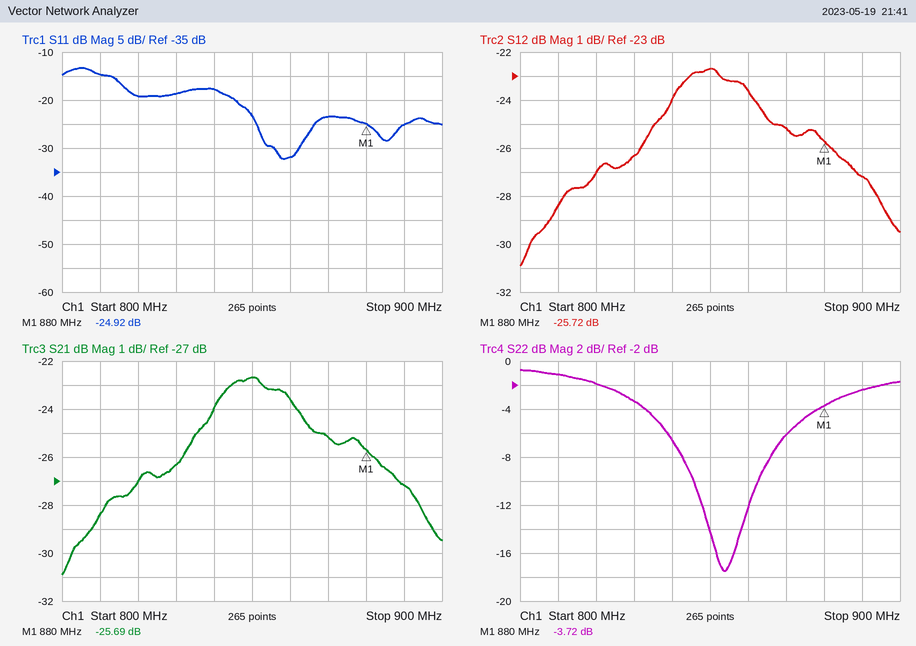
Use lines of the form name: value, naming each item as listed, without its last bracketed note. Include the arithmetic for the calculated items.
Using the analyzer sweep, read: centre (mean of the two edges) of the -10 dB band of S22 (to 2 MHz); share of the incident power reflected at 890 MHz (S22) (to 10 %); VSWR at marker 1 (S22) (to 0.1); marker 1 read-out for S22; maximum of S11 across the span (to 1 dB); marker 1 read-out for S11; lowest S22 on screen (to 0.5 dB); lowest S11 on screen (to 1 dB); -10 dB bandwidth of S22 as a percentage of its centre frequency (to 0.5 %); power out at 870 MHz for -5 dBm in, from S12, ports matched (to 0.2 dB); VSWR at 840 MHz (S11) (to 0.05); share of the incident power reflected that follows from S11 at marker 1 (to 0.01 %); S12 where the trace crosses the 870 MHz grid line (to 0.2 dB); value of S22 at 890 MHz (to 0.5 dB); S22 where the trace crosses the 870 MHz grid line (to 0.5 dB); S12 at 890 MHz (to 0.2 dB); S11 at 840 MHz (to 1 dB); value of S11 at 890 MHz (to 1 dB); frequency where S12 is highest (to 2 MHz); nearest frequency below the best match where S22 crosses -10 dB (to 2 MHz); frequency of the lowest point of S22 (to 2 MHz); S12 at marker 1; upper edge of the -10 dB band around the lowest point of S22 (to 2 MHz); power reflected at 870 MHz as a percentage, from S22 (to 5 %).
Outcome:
centre (mean of the two edges) of the -10 dB band of S22: 854 MHz
share of the incident power reflected at 890 MHz (S22): 10^(-2.5/10) ≈ 56.2 %, so 60 % to the nearest 10 %
VSWR at marker 1 (S22): (1 + 0.6516)/(1 − 0.6516) ≈ 4.7
marker 1 read-out for S22: -3.72 dB
maximum of S11 across the span: -13 dB
marker 1 read-out for S11: -24.92 dB
lowest S22 on screen: -17.5 dB
lowest S11 on screen: -32 dB
-10 dB bandwidth of S22 as a percentage of its centre frequency: 16 MHz / 854 MHz ≈ 1.87 %, so 2.0 % to the nearest 0.5 %
power out at 870 MHz for -5 dBm in, from S12, ports matched: -5 dBm + (-25.2 dB) = -30.2 dBm
VSWR at 840 MHz (S11): |Γ| = 10^(-18/20) = 0.1259; VSWR = (1 + 0.1259)/(1 − 0.1259) ≈ 1.29, so 1.30 to the nearest 0.05
share of the incident power reflected that follows from S11 at marker 1: 10^(-24.92/10) ≈ 0.32 %
S12 where the trace crosses the 870 MHz grid line: -25.2 dB
value of S22 at 890 MHz: -2.5 dB
S22 where the trace crosses the 870 MHz grid line: -6.0 dB
S12 at 890 MHz: -27.2 dB
S11 at 840 MHz: -18 dB
value of S11 at 890 MHz: -25 dB
frequency where S12 is highest: 850 MHz
nearest frequency below the best match where S22 crosses -10 dB: 846 MHz
frequency of the lowest point of S22: 854 MHz
S12 at marker 1: -25.72 dB
upper edge of the -10 dB band around the lowest point of S22: 862 MHz
power reflected at 870 MHz as a percentage, from S22: 10^(-6/10) ≈ 25 %
